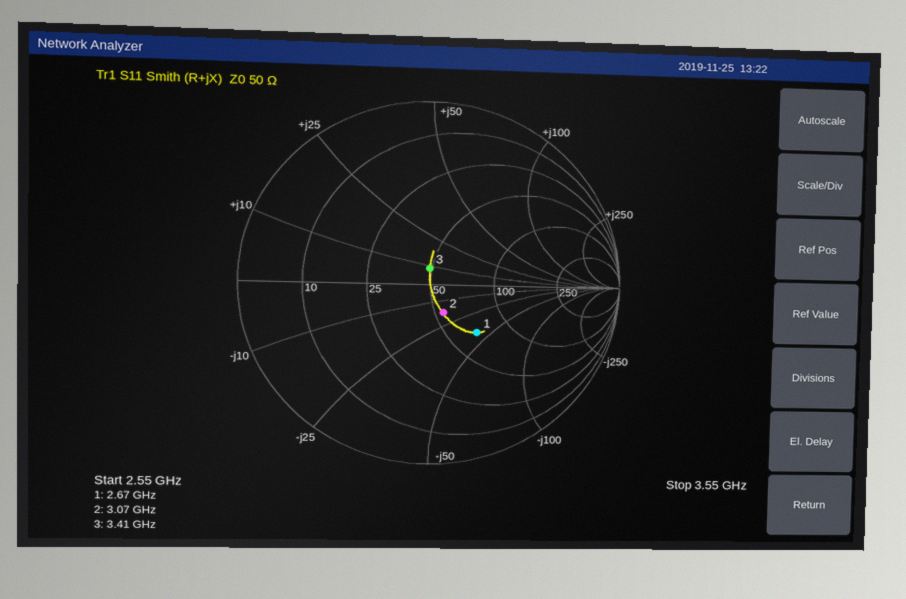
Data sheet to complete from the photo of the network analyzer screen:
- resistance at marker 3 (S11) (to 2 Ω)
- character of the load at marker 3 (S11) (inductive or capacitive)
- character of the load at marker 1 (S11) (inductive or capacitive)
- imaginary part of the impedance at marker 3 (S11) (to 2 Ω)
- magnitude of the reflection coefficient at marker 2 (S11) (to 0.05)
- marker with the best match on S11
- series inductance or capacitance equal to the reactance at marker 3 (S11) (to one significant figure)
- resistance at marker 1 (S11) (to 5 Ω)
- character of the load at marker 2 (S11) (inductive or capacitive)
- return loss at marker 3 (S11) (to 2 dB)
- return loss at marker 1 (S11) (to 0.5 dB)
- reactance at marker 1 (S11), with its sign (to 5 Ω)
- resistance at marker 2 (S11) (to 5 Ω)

48 Ω
inductive
capacitive
+8 Ω
0.15
marker 3
400 pH
70 Ω
capacitive
22 dB
9.0 dB
-40 Ω
55 Ω
